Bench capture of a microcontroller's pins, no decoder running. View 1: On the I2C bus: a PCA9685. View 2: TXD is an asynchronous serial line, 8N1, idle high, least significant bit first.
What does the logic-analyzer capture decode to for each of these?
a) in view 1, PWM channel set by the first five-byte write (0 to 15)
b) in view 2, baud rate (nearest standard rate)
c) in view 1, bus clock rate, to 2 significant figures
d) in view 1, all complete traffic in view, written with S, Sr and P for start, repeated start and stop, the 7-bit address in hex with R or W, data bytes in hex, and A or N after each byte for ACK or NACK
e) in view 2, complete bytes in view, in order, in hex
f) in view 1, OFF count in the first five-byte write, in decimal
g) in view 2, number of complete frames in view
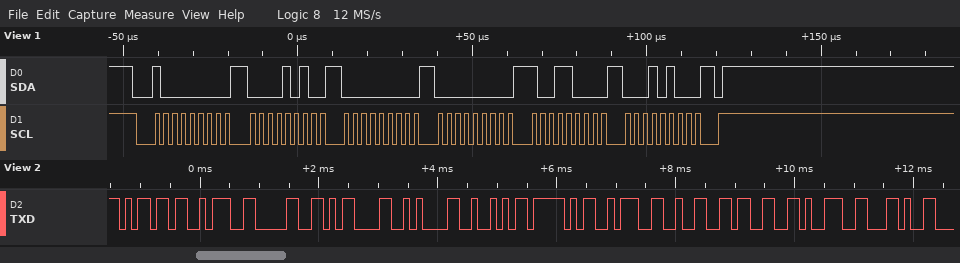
1
9600 baud
400 kHz
S 40W A 0A A 00 A 00 A 98 A 14 A P
6D 3A 30 0D 0A 52 5F 3A 32 33 39 2C
5272
12
